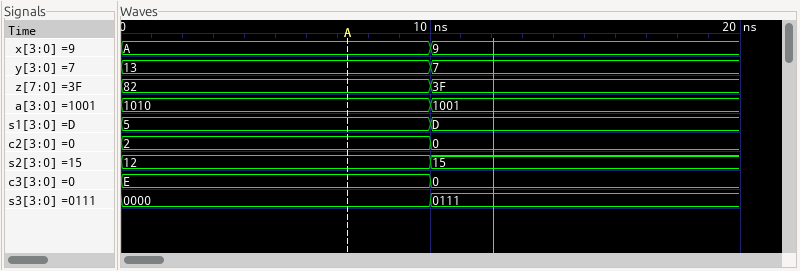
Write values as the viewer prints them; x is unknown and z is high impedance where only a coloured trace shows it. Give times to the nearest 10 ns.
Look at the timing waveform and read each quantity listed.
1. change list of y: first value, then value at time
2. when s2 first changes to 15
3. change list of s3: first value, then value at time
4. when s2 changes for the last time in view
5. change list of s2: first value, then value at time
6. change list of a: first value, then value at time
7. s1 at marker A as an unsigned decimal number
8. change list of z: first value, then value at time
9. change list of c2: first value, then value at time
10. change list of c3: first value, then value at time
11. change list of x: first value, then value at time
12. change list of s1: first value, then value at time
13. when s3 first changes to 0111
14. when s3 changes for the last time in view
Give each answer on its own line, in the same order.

13, 7 at 10 ns
10 ns
0000, 0111 at 10 ns
10 ns
12, 15 at 10 ns
1010, 1001 at 10 ns
5
82, 3F at 10 ns
2, 0 at 10 ns
E, 0 at 10 ns
A, 9 at 10 ns
5, D at 10 ns
10 ns
10 ns
